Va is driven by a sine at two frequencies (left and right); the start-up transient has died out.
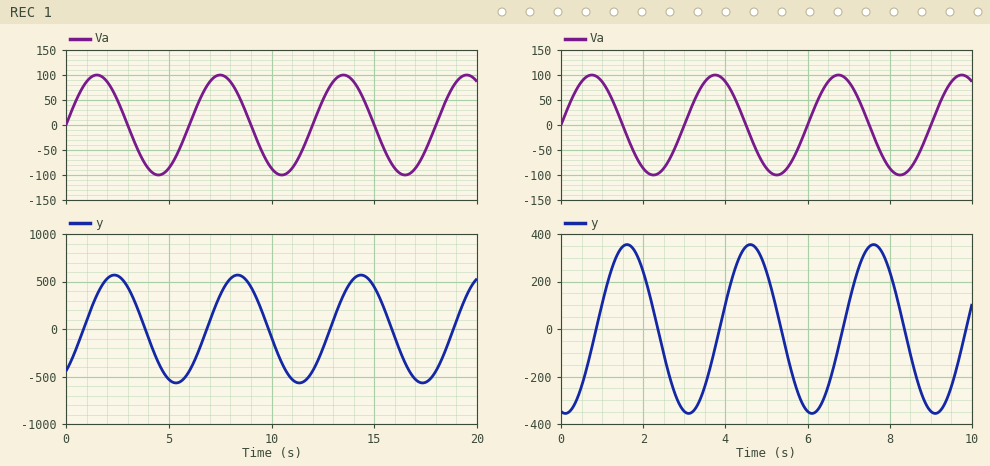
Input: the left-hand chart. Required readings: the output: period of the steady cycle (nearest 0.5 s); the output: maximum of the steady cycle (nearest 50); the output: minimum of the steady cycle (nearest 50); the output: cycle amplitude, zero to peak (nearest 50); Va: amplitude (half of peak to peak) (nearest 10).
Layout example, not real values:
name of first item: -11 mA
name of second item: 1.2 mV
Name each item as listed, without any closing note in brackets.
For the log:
the output: period of the steady cycle: 6.0 s
the output: maximum of the steady cycle: 550
the output: minimum of the steady cycle: -550
the output: cycle amplitude, zero to peak: 550
Va: amplitude (half of peak to peak): 100
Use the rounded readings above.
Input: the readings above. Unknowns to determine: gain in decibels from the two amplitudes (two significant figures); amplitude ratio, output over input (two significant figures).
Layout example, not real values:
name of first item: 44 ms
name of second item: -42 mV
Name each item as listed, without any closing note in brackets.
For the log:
gain in decibels from the two amplitudes: 15 dB
amplitude ratio, output over input: 5.5
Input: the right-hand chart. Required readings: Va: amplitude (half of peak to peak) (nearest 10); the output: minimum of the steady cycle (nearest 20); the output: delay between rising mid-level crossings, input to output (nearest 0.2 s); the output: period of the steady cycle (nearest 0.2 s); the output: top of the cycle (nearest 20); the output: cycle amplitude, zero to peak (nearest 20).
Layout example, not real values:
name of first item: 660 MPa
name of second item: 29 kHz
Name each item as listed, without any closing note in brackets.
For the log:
Va: amplitude (half of peak to peak): 100
the output: minimum of the steady cycle: -360
the output: delay between rising mid-level crossings, input to output: 0.8 s
the output: period of the steady cycle: 3.0 s
the output: top of the cycle: 360
the output: cycle amplitude, zero to peak: 360
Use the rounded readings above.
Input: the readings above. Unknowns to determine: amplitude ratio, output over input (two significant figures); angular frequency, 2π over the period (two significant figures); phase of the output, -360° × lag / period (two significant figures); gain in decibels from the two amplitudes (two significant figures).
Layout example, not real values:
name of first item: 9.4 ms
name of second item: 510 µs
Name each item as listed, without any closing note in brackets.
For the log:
amplitude ratio, output over input: 3.6
angular frequency, 2π over the period: 2.1 rad/s
phase of the output, -360° × lag / period: -96°
gain in decibels from the two amplitudes: 11 dB
